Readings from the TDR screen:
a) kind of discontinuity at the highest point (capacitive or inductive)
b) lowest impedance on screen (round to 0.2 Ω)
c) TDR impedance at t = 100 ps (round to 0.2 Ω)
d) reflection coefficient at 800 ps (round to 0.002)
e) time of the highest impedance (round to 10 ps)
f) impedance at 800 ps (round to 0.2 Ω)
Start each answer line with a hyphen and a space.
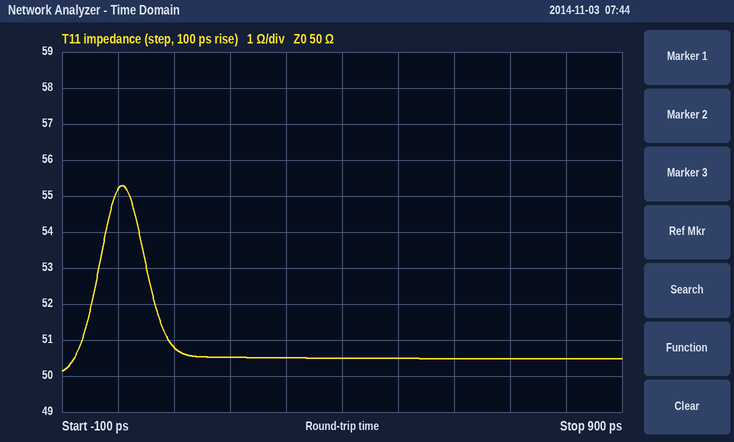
- inductive
- 50.2 Ω
- 50.8 Ω
- +0.004
- 10 ps
- 50.4 Ω
